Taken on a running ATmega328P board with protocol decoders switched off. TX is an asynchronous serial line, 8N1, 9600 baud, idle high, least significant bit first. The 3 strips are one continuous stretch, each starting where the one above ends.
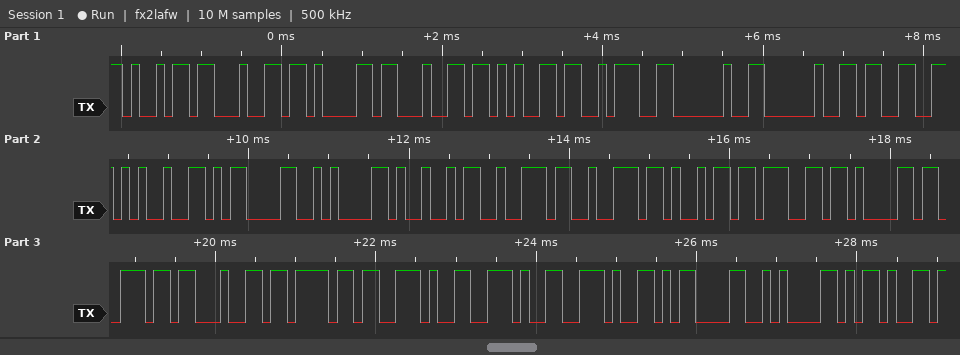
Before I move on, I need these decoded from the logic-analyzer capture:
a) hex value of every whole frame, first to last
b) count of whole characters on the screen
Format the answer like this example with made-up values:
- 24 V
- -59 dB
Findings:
- 69 64 61 64 65 3A 20 20 33 25 0D 0A 49 72 72 69 67 61 6E 64 6F 2E 2E 2E 0D 0A 2D
- 27
